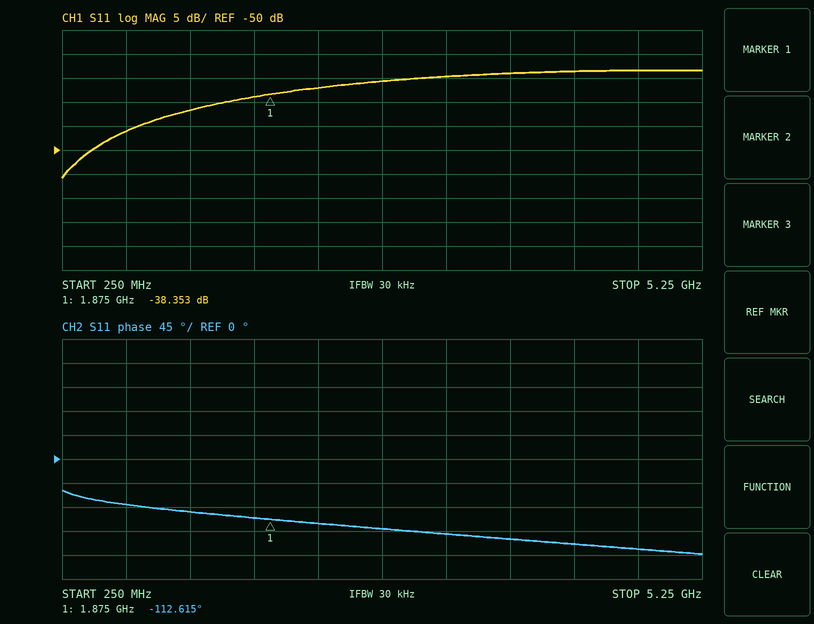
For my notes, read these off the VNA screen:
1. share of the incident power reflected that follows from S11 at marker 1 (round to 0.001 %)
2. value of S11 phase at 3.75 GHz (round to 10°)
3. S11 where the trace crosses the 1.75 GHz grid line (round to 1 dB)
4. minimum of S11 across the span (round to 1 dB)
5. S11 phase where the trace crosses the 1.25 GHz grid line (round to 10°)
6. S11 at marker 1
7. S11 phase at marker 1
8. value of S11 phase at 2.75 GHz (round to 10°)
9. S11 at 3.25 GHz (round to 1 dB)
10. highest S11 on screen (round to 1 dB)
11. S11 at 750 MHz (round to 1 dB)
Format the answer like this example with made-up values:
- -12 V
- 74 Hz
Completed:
- 0.015 %
- -150°
- -39 dB
- -56 dB
- -100°
- -38.353 dB
- -112.615°
- -130°
- -35 dB
- -33 dB
- -46 dB
